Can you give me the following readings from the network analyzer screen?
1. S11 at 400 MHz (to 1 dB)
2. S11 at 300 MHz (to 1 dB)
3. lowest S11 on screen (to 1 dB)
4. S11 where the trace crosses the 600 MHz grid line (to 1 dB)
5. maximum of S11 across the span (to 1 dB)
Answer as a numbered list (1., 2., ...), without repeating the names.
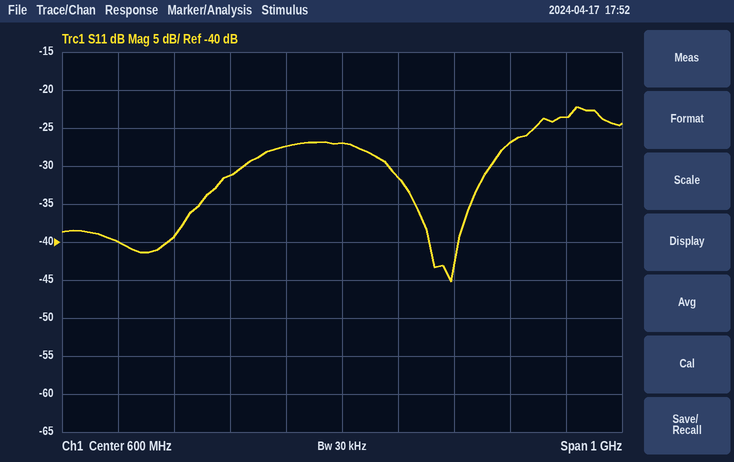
1. -31 dB
2. -39 dB
3. -45 dB
4. -27 dB
5. -22 dB
